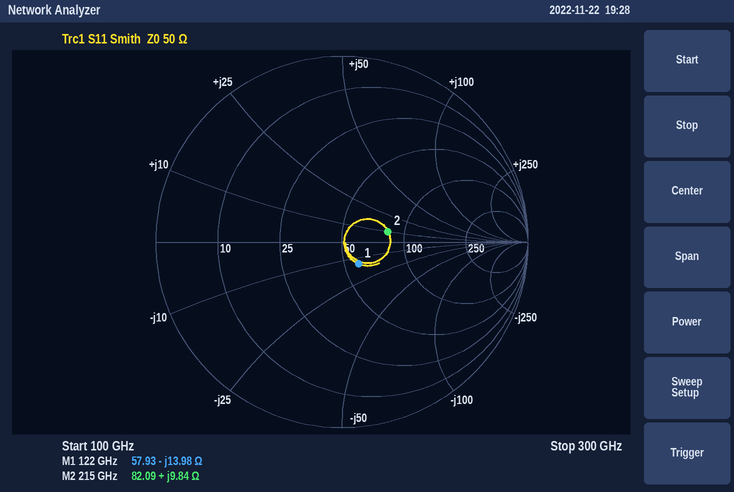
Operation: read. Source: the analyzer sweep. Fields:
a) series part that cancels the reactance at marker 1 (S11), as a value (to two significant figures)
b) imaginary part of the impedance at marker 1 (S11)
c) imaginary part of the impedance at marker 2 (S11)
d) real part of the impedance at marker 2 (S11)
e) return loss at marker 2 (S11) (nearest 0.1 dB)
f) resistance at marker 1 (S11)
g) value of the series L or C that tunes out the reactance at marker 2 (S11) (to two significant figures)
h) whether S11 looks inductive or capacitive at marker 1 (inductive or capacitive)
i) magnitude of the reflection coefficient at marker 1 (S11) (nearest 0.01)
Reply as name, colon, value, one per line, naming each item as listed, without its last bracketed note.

series part that cancels the reactance at marker 1 (S11), as a value: 18 pH
imaginary part of the impedance at marker 1: -13.98 Ω
imaginary part of the impedance at marker 2: +9.84 Ω
real part of the impedance at marker 2: 82.09 Ω
return loss at marker 2 (S11): 11.9 dB
resistance at marker 1: 57.93 Ω
value of the series L or C that tunes out the reactance at marker 2 (S11): 75 fF
whether S11 looks inductive or capacitive at marker 1: capacitive
magnitude of the reflection coefficient at marker 1 (S11): 0.15
